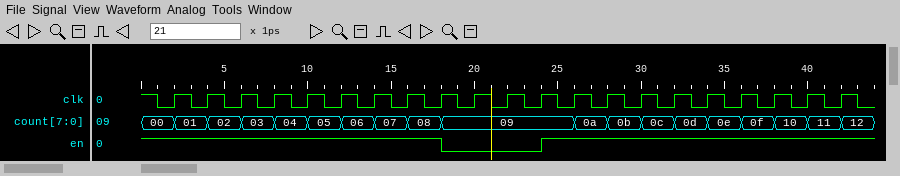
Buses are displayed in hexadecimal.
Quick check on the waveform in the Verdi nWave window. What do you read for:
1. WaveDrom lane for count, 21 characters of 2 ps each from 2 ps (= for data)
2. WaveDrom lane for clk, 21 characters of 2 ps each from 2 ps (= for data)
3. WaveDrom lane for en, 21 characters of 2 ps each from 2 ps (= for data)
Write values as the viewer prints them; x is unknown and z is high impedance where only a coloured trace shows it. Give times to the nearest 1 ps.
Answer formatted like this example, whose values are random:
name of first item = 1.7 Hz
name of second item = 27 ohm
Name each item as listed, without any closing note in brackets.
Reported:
WaveDrom lane for count, 21 characters of 2 ps each from 2 ps = {name: 'count', wave: '=========...=========', data: '01 02 03 04 05 06 07 08 09 0a 0b 0c 0d 0e 0f 10 11 12'}
WaveDrom lane for clk, 21 characters of 2 ps each from 2 ps = {name: 'clk', wave: 'p....................'}
WaveDrom lane for en, 21 characters of 2 ps each from 2 ps = {name: 'en', wave: '1.......0..1.........'}
